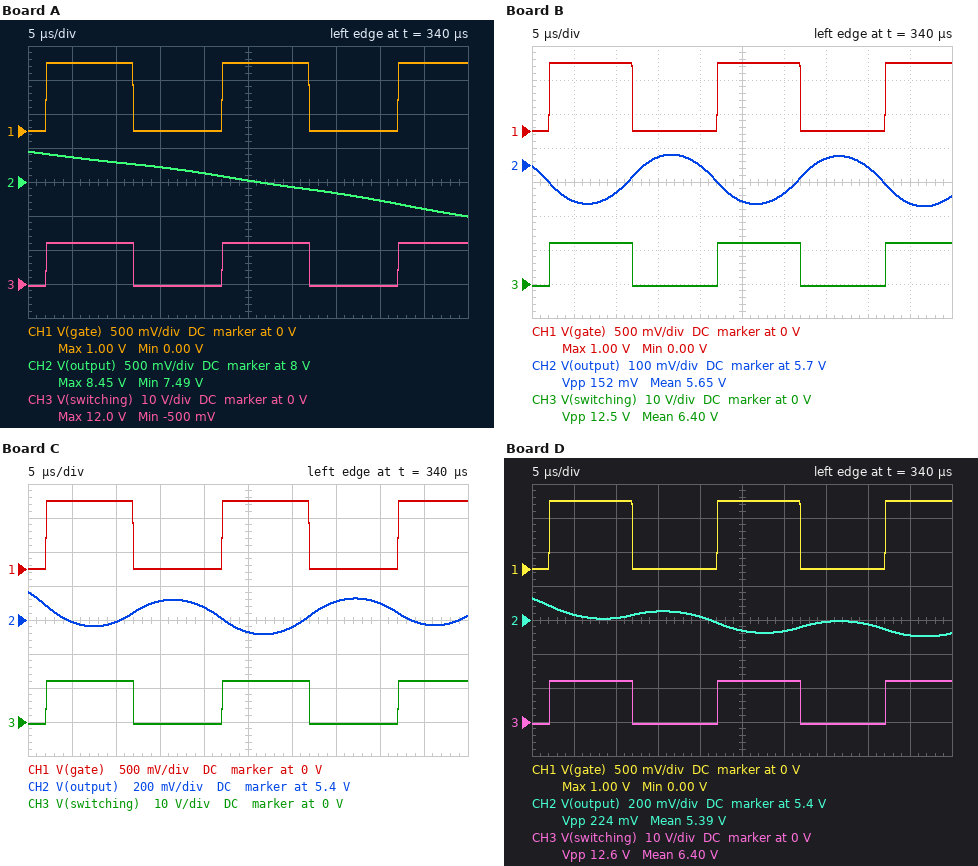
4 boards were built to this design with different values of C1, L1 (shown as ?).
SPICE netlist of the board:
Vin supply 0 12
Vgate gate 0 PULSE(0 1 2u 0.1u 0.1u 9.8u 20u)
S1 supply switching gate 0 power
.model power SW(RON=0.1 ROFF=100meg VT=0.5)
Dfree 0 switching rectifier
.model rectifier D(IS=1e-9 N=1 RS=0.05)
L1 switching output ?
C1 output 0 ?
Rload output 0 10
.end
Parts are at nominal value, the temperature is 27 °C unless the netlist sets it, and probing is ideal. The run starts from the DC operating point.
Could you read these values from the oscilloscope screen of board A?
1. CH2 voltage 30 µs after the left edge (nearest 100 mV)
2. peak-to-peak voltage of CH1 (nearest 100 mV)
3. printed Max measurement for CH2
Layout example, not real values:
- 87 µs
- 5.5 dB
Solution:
- 7.9 V
- 1.0 V
- 8.45 V
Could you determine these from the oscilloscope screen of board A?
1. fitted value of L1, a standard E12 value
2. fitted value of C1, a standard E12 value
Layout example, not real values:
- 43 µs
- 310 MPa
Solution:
- 330 µH
- 27 µF
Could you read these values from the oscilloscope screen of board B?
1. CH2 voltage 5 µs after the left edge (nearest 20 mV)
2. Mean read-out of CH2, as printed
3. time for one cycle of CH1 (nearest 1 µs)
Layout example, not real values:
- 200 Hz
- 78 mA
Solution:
- 5.60 V
- 5.65 V
- 20 µs
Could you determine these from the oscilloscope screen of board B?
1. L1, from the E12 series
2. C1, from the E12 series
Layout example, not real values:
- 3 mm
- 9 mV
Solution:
- 330 µH
- 3.3 µF
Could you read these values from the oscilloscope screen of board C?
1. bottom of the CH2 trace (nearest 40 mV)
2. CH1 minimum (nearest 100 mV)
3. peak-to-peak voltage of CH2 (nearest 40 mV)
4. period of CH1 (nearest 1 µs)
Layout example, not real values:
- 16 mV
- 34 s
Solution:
- 5.32 V
- 0 V
- 240 mV
- 20 µs
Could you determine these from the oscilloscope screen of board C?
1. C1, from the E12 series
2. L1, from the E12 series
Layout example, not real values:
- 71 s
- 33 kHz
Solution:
- 6.8 µF
- 120 µH
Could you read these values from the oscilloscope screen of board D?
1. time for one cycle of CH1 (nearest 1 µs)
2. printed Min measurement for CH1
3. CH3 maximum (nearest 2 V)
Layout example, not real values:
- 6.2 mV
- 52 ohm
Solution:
- 20 µs
- 0.00 V
- 12 V
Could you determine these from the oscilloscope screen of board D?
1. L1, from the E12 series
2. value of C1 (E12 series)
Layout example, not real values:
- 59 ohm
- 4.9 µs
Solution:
- 82 µH
- 22 µF
